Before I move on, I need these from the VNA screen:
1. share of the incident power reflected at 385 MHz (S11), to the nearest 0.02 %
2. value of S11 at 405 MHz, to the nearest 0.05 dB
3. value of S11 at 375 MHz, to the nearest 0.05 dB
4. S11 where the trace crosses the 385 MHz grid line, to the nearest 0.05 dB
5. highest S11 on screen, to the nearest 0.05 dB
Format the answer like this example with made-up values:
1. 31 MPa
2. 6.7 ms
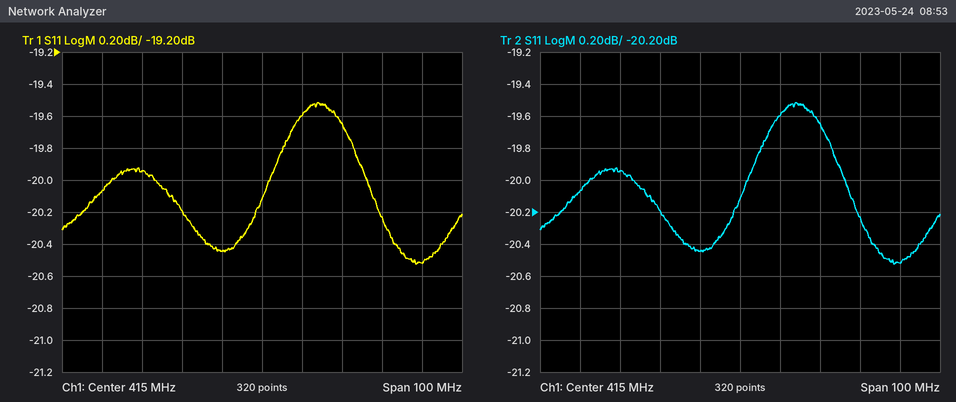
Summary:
1. 1.02 %
2. -20.45 dB
3. -20.05 dB
4. -19.95 dB
5. -19.50 dB
